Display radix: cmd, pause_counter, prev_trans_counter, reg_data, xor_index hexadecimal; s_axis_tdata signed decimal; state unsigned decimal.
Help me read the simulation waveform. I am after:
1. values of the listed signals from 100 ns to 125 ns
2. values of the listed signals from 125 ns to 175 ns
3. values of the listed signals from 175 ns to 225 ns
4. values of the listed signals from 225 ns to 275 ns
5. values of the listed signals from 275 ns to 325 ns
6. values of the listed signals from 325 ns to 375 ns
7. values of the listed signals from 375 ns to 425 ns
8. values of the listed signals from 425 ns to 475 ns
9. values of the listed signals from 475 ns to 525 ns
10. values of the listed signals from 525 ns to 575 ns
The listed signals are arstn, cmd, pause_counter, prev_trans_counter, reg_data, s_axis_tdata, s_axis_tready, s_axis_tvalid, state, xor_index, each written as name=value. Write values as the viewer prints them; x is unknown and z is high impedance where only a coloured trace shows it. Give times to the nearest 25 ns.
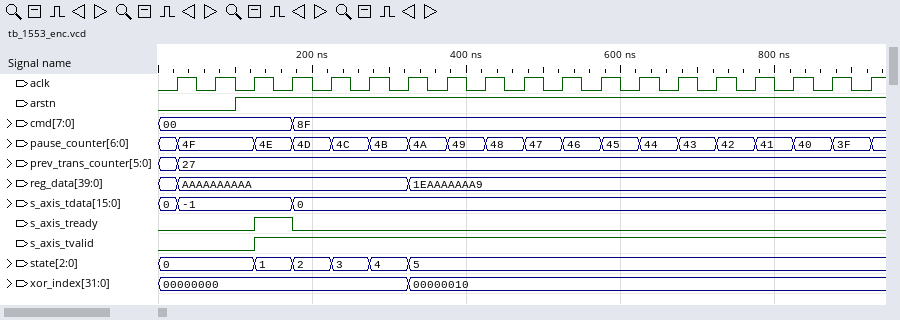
arstn=1, cmd=00, pause_counter=4F, prev_trans_counter=27, reg_data=AAAAAAAAAA, s_axis_tdata=-1, s_axis_tready=0, s_axis_tvalid=0, state=0, xor_index=00000000
arstn=1, cmd=00, pause_counter=4E, prev_trans_counter=27, reg_data=AAAAAAAAAA, s_axis_tdata=-1, s_axis_tready=1, s_axis_tvalid=1, state=1, xor_index=00000000
arstn=1, cmd=8F, pause_counter=4D, prev_trans_counter=27, reg_data=AAAAAAAAAA, s_axis_tdata=0, s_axis_tready=0, s_axis_tvalid=1, state=2, xor_index=00000000
arstn=1, cmd=8F, pause_counter=4C, prev_trans_counter=27, reg_data=AAAAAAAAAA, s_axis_tdata=0, s_axis_tready=0, s_axis_tvalid=1, state=3, xor_index=00000000
arstn=1, cmd=8F, pause_counter=4B, prev_trans_counter=27, reg_data=AAAAAAAAAA, s_axis_tdata=0, s_axis_tready=0, s_axis_tvalid=1, state=4, xor_index=00000000
arstn=1, cmd=8F, pause_counter=4A, prev_trans_counter=27, reg_data=1EAAAAAAA9, s_axis_tdata=0, s_axis_tready=0, s_axis_tvalid=1, state=5, xor_index=00000010
arstn=1, cmd=8F, pause_counter=49, prev_trans_counter=27, reg_data=1EAAAAAAA9, s_axis_tdata=0, s_axis_tready=0, s_axis_tvalid=1, state=5, xor_index=00000010
arstn=1, cmd=8F, pause_counter=48, prev_trans_counter=27, reg_data=1EAAAAAAA9, s_axis_tdata=0, s_axis_tready=0, s_axis_tvalid=1, state=5, xor_index=00000010
arstn=1, cmd=8F, pause_counter=47, prev_trans_counter=27, reg_data=1EAAAAAAA9, s_axis_tdata=0, s_axis_tready=0, s_axis_tvalid=1, state=5, xor_index=00000010
arstn=1, cmd=8F, pause_counter=46, prev_trans_counter=27, reg_data=1EAAAAAAA9, s_axis_tdata=0, s_axis_tready=0, s_axis_tvalid=1, state=5, xor_index=00000010
